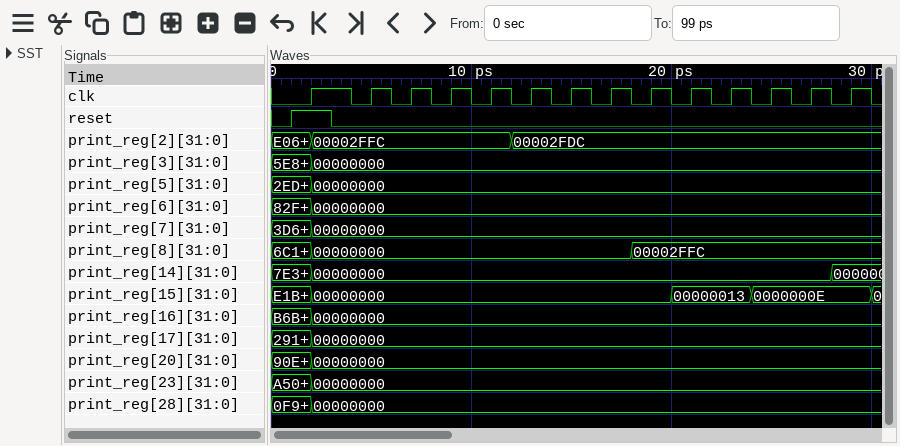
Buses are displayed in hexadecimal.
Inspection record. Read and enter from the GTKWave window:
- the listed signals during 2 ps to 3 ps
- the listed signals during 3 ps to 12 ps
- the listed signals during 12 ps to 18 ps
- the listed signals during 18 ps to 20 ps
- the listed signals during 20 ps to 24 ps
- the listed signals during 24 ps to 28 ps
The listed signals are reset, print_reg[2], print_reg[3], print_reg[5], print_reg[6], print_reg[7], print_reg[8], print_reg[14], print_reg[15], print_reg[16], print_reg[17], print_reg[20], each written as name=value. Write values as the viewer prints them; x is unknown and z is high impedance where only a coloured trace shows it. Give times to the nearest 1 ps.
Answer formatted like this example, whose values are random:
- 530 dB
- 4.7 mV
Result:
- reset=1, print_reg[2]=00002FFC, print_reg[3]=00000000, print_reg[5]=00000000, print_reg[6]=00000000, print_reg[7]=00000000, print_reg[8]=00000000, print_reg[14]=00000000, print_reg[15]=00000000, print_reg[16]=00000000, print_reg[17]=00000000, print_reg[20]=00000000
- reset=0, print_reg[2]=00002FFC, print_reg[3]=00000000, print_reg[5]=00000000, print_reg[6]=00000000, print_reg[7]=00000000, print_reg[8]=00000000, print_reg[14]=00000000, print_reg[15]=00000000, print_reg[16]=00000000, print_reg[17]=00000000, print_reg[20]=00000000
- reset=0, print_reg[2]=00002FDC, print_reg[3]=00000000, print_reg[5]=00000000, print_reg[6]=00000000, print_reg[7]=00000000, print_reg[8]=00000000, print_reg[14]=00000000, print_reg[15]=00000000, print_reg[16]=00000000, print_reg[17]=00000000, print_reg[20]=00000000
- reset=0, print_reg[2]=00002FDC, print_reg[3]=00000000, print_reg[5]=00000000, print_reg[6]=00000000, print_reg[7]=00000000, print_reg[8]=00002FFC, print_reg[14]=00000000, print_reg[15]=00000000, print_reg[16]=00000000, print_reg[17]=00000000, print_reg[20]=00000000
- reset=0, print_reg[2]=00002FDC, print_reg[3]=00000000, print_reg[5]=00000000, print_reg[6]=00000000, print_reg[7]=00000000, print_reg[8]=00002FFC, print_reg[14]=00000000, print_reg[15]=00000013, print_reg[16]=00000000, print_reg[17]=00000000, print_reg[20]=00000000
- reset=0, print_reg[2]=00002FDC, print_reg[3]=00000000, print_reg[5]=00000000, print_reg[6]=00000000, print_reg[7]=00000000, print_reg[8]=00002FFC, print_reg[14]=00000000, print_reg[15]=0000000E, print_reg[16]=00000000, print_reg[17]=00000000, print_reg[20]=00000000
